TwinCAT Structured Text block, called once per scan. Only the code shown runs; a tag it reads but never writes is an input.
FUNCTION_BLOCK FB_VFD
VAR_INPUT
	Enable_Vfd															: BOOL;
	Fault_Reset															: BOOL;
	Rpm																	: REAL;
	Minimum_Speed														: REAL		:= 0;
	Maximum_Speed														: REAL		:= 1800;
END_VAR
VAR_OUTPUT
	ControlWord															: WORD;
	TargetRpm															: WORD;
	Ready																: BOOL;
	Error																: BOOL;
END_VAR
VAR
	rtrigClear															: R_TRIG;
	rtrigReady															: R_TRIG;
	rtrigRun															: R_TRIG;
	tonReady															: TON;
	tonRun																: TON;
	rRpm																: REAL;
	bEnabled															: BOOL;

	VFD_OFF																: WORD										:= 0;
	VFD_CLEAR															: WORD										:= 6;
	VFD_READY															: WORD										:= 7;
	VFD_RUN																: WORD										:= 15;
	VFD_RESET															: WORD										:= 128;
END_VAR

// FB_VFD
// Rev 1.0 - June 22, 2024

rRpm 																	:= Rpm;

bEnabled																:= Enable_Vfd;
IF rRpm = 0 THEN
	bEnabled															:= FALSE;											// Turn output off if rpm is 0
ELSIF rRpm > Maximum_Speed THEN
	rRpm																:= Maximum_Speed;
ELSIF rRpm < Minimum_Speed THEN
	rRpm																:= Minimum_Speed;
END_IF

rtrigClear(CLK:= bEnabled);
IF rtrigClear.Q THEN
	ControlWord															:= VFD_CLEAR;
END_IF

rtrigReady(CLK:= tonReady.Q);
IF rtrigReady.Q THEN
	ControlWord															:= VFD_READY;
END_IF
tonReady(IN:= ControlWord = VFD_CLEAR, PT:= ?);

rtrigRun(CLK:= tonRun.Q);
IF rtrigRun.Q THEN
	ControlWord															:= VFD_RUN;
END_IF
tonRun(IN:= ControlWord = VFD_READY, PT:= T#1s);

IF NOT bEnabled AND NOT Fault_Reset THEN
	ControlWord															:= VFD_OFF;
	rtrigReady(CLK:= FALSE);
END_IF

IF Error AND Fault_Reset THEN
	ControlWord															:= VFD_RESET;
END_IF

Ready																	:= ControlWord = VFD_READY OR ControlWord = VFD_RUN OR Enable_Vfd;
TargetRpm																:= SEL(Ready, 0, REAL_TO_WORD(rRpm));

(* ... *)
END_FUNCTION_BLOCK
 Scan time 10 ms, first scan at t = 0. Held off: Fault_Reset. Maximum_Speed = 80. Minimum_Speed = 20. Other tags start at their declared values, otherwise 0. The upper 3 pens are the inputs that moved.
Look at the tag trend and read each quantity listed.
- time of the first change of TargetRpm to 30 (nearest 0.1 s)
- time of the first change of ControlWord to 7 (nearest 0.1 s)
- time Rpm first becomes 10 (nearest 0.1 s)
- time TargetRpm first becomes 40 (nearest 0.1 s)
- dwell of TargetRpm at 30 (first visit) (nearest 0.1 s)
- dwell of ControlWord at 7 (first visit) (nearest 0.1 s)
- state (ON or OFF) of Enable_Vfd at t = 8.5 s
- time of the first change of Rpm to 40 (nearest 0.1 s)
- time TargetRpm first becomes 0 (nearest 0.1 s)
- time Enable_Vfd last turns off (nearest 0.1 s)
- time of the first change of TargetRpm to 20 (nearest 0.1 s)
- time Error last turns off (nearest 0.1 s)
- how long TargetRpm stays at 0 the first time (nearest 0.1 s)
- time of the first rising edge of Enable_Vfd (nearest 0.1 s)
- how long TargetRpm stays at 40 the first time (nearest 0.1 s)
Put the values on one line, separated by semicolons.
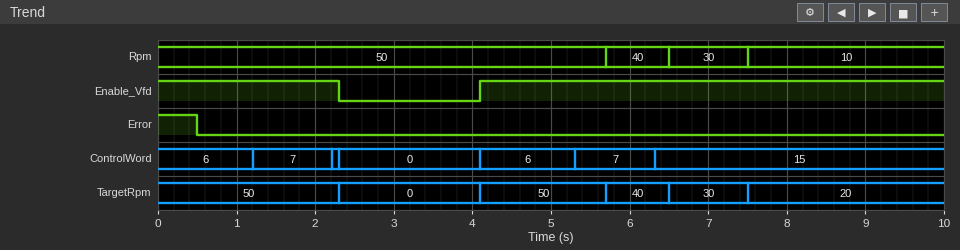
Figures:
6.5 s; 1.2 s; 7.5 s; 5.7 s; 1.0 s; 1.0 s; ON; 5.7 s; 2.3 s; 2.3 s; 7.5 s; 0.5 s; 1.8 s; 4.1 s; 0.8 s
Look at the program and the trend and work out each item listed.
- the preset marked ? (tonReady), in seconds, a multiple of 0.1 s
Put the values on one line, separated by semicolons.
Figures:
1.2 s
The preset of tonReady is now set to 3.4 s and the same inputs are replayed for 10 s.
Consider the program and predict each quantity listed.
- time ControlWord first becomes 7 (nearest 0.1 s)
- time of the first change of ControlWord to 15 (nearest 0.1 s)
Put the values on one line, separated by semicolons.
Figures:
7.5 s; 8.5 s
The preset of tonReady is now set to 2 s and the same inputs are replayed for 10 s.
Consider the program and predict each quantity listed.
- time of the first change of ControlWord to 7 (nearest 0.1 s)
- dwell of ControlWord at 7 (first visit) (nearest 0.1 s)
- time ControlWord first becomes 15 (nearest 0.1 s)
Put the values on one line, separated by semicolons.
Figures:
2.0 s; 0.3 s; 7.1 s
